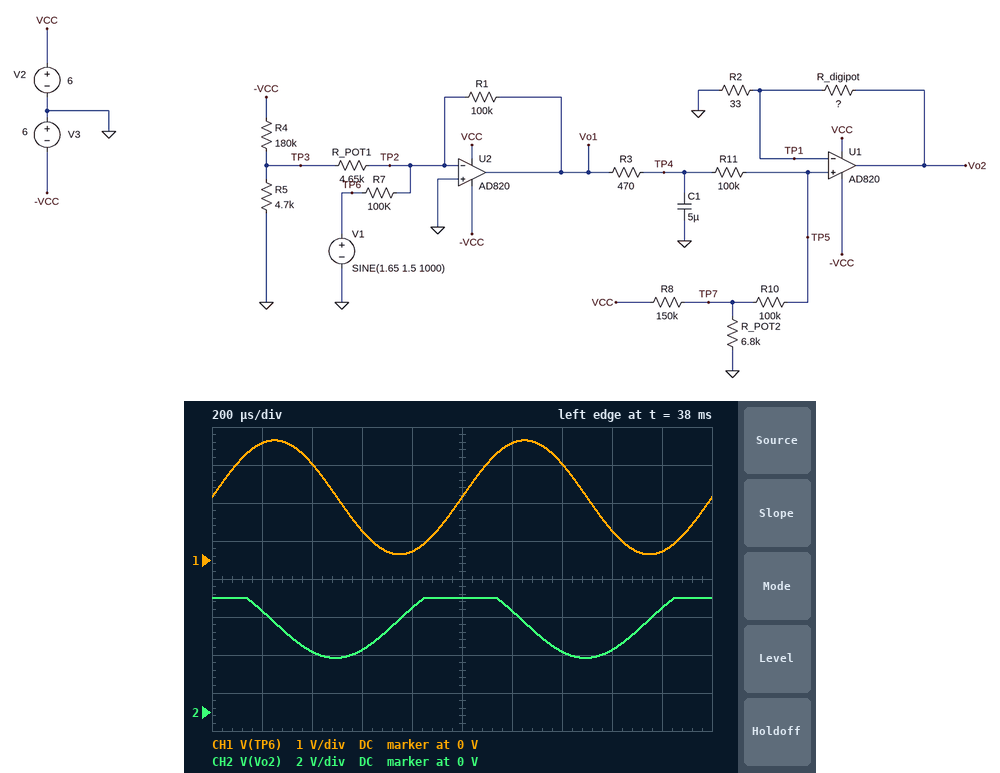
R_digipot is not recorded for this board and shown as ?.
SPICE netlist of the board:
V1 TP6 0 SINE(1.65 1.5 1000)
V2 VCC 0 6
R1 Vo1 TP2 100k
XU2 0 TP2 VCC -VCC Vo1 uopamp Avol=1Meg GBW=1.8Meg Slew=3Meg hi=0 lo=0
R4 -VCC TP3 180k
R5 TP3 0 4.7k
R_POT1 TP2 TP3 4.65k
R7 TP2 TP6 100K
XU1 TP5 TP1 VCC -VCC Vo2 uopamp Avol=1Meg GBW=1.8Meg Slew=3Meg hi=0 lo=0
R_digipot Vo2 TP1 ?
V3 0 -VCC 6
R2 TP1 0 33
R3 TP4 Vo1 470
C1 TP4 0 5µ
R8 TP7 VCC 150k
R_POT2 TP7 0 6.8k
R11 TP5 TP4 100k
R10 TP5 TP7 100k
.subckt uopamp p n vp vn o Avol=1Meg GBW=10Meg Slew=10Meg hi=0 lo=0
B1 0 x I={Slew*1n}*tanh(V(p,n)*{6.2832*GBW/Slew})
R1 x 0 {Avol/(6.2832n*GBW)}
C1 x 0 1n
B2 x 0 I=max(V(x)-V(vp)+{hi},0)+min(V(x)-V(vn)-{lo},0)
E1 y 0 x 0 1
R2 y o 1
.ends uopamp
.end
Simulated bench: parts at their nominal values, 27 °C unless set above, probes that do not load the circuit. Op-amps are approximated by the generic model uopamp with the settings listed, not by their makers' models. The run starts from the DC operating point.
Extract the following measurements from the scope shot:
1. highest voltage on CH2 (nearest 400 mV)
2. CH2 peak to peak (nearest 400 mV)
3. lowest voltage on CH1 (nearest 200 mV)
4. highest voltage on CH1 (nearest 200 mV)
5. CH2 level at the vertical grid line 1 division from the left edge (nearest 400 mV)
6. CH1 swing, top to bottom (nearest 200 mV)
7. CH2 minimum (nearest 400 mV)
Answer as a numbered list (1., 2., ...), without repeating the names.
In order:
1. 6.0 V
2. 3.2 V
3. 200 mV
4. 3.2 V
5. 5.2 V
6. 3.0 V
7. 2.8 V
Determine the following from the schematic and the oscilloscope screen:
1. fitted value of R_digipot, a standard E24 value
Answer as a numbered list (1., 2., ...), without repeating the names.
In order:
1. 1.2 kΩ
